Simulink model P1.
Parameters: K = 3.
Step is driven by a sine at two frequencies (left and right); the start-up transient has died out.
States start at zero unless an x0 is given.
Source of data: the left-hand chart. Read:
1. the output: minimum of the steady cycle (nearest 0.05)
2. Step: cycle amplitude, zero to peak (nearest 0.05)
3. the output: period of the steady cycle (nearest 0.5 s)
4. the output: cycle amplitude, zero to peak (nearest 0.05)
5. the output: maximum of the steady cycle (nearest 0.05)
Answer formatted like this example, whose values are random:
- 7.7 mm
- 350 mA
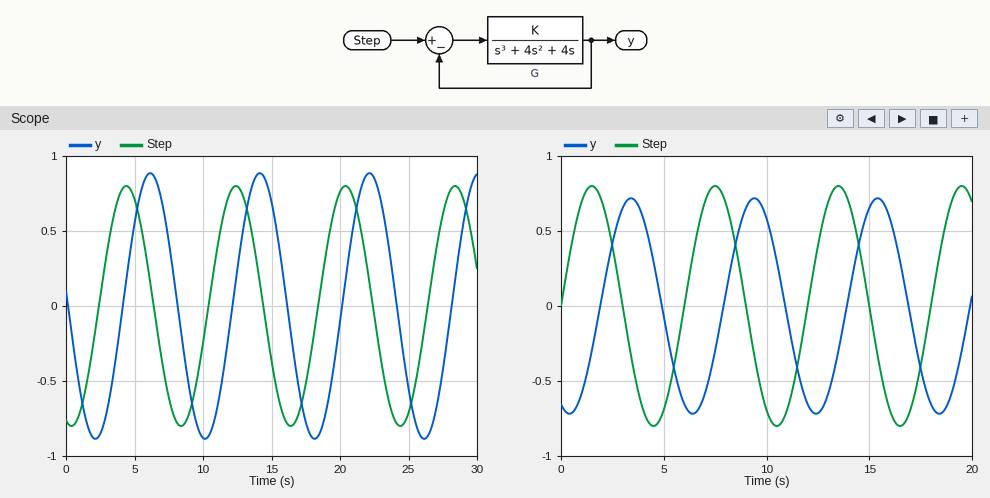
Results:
- -0.90
- 0.80
- 8.0 s
- 0.90
- 0.90
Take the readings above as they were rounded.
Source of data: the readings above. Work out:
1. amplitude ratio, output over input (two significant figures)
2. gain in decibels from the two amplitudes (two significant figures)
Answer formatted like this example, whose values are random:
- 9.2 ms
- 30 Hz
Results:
- 1.1
- 1.0 dB
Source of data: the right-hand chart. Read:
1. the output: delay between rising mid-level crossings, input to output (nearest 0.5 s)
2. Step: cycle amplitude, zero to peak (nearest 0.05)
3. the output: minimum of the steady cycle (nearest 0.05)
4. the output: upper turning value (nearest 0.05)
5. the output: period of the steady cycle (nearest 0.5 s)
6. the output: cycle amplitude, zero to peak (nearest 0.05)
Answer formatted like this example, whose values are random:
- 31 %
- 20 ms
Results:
- 2.0 s
- 0.80
- -0.70
- 0.70
- 6.0 s
- 0.70
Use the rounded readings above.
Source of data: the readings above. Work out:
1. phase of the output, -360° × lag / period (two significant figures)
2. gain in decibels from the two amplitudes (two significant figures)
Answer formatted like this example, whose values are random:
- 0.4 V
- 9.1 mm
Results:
- -120°
- -1.2 dB
